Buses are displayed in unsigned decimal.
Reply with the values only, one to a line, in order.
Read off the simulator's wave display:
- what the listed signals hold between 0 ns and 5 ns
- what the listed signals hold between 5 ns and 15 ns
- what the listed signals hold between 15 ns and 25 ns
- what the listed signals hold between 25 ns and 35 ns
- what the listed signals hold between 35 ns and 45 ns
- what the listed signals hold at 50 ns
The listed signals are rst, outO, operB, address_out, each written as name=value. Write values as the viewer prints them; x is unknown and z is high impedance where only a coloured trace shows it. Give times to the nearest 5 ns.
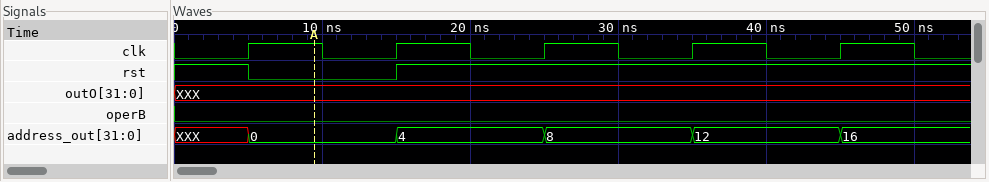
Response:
rst=1, outO=XXX, operB=0, address_out=XXX
rst=0, outO=XXX, operB=0, address_out=0
rst=1, outO=XXX, operB=0, address_out=4
rst=1, outO=XXX, operB=0, address_out=8
rst=1, outO=XXX, operB=0, address_out=12
rst=1, outO=XXX, operB=0, address_out=16
